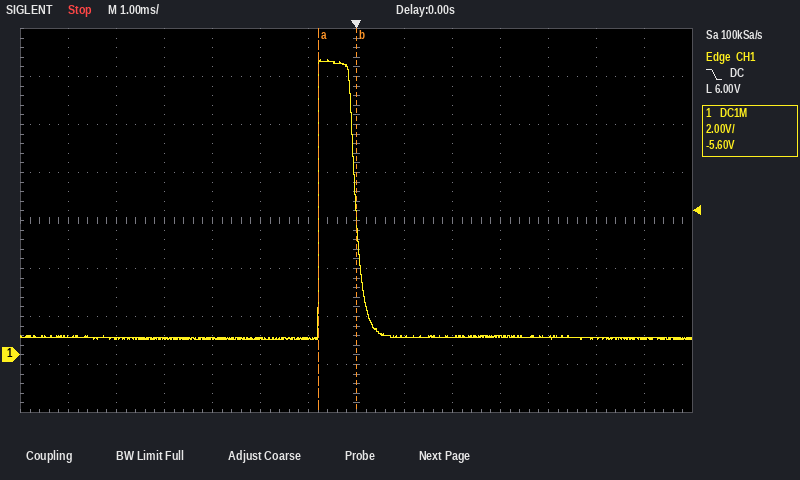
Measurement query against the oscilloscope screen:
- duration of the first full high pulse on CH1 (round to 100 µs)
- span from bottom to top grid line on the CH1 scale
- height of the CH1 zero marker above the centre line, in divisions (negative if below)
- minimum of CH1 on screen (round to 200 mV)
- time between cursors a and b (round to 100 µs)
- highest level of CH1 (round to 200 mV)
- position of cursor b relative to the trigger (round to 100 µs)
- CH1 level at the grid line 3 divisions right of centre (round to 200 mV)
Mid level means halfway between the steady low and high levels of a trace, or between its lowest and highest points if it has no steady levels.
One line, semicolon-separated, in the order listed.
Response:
800 µs; 16 V; -2.8 div; 600 mV; 800 µs; 12.4 V; 0.0 ms; 800 mV
